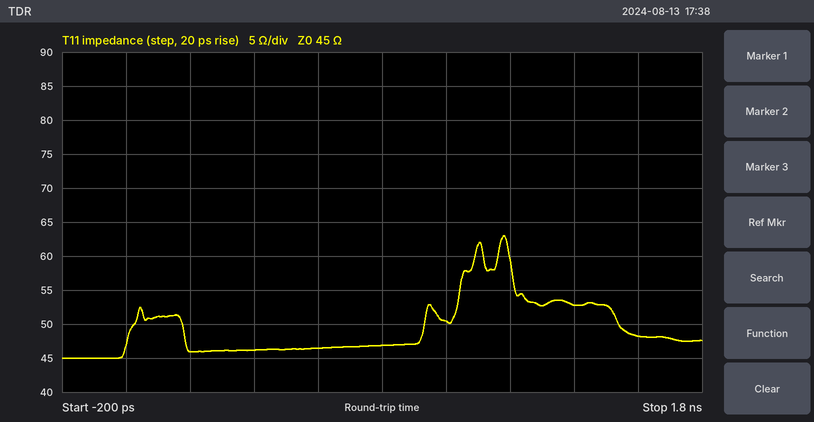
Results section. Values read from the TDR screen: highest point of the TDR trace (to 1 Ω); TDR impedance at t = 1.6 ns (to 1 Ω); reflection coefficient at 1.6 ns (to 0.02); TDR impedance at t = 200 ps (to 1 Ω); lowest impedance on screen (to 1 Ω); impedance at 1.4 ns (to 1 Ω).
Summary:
63 Ω
48 Ω
+0.04
46 Ω
45 Ω
53 Ω
